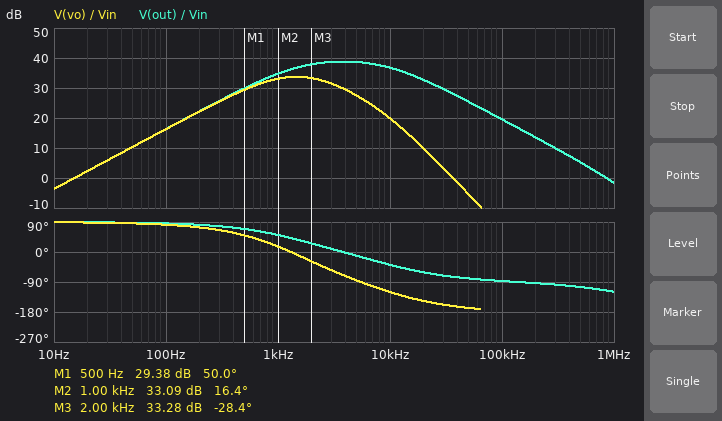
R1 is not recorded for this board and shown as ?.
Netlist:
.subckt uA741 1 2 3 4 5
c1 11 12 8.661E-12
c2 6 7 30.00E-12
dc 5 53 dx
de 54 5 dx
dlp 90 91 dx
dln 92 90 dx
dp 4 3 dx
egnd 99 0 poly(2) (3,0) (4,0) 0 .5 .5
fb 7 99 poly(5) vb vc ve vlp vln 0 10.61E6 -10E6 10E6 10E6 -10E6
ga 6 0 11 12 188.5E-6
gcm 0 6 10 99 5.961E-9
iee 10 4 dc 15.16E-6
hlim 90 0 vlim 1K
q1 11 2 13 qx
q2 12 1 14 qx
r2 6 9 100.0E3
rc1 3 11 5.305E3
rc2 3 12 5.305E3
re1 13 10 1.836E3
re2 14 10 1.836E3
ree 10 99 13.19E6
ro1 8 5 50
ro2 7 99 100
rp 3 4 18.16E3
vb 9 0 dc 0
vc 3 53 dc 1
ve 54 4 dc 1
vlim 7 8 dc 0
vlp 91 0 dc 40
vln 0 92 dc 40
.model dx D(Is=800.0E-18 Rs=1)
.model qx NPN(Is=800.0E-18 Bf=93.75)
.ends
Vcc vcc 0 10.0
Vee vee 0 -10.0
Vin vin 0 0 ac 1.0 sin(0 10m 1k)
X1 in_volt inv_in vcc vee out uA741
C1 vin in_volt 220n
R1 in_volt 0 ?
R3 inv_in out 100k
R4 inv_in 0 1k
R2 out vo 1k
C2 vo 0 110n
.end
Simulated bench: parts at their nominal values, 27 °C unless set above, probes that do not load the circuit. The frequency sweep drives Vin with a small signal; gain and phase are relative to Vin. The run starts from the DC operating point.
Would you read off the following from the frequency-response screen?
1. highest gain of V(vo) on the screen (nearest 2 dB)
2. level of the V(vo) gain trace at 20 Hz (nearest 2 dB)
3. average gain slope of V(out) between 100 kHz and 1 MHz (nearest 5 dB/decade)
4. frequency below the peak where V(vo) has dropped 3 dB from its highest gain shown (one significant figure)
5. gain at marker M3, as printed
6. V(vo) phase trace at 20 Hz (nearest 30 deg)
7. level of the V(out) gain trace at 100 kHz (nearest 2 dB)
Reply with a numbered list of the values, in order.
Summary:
1. 34 dB
2. 2 dB
3. -20 dB/decade
4. 600 Hz
5. 33.28 dB
6. 90 deg
7. 20 dB
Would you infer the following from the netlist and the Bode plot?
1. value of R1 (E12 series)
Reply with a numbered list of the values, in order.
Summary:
1. 470 Ω
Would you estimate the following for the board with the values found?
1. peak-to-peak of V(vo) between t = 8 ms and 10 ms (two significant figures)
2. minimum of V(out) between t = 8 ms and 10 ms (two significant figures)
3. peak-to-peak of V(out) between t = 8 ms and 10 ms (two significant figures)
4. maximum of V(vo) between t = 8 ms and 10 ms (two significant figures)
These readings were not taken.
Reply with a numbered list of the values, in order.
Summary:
1. 900 mV
2. -540 mV
3. 1.1 V
4. 460 mV
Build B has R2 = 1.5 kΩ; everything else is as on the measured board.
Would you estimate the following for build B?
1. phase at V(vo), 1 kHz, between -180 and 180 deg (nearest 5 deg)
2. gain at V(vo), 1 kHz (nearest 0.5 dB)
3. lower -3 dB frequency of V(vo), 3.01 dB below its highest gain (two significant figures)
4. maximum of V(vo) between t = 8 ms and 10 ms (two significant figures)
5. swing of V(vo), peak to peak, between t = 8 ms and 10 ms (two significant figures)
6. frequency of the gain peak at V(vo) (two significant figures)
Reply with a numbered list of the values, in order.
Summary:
1. 5 deg
2. 31.5 dB
3. 490 Hz
4. 390 mV
5. 760 mV
6. 1.2 kHz
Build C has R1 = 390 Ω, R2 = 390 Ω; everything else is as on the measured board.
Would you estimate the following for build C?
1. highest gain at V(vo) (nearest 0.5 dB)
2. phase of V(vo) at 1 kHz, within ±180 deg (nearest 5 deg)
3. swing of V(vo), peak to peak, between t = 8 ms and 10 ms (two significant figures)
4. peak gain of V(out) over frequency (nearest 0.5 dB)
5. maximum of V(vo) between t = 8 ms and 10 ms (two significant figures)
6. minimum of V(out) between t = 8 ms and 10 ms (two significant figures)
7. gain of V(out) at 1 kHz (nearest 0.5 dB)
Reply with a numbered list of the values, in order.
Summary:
1. 36.5 dB
2. 40 deg
3. 920 mV
4. 38.5 dB
5. 470 mV
6. -470 mV
7. 33.5 dB
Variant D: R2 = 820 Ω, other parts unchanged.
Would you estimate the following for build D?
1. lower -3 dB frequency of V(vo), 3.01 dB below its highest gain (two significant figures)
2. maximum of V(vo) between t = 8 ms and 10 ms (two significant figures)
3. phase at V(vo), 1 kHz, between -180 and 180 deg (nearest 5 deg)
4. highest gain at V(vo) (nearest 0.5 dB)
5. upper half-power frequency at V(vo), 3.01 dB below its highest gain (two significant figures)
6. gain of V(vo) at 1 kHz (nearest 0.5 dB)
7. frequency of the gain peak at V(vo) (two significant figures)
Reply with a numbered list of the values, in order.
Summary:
1. 670 Hz
2. 480 mV
3. 20 deg
4. 34.5 dB
5. 3.7 kHz
6. 33.5 dB
7. 1.6 kHz
